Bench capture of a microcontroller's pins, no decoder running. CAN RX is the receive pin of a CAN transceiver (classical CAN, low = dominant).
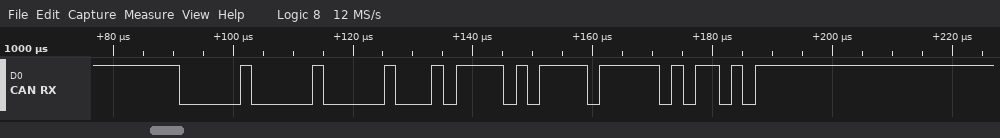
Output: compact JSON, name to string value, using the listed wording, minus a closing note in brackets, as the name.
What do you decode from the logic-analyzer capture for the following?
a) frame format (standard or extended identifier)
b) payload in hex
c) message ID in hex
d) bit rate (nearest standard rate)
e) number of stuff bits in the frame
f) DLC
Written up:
{"frame format": "standard", "payload in hex": "7A", "message ID in hex": "0x000", "bit rate": "500 kbit/s", "number of stuff bits in the frame": "4", "DLC": "1"}
